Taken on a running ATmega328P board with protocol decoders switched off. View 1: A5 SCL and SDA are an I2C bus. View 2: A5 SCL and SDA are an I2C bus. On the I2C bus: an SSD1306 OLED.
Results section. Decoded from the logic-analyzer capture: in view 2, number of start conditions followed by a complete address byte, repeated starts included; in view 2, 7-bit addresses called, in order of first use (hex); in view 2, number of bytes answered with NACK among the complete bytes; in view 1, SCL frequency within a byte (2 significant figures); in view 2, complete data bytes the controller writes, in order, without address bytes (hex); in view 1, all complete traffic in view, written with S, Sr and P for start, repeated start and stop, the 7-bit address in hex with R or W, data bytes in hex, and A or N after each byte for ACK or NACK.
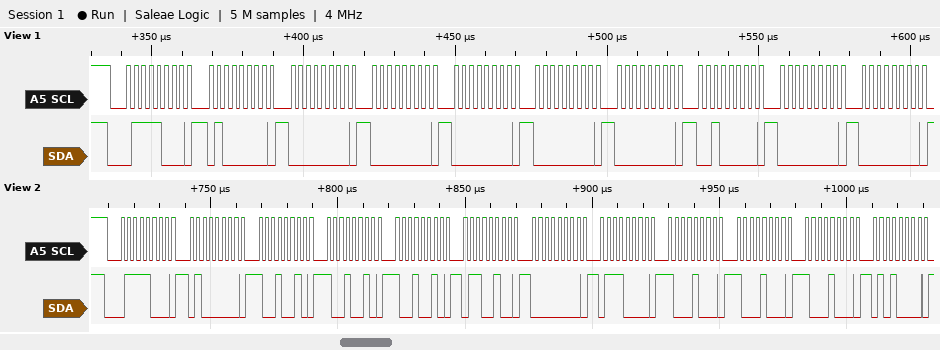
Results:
1
0x3C
0
400 kHz
40 92 92 92 64 00 70 88 88 88 50
S 3CW A 40 A 00 A 00 A 00 A 00 A 00 A 20 A 00 A 00 A
